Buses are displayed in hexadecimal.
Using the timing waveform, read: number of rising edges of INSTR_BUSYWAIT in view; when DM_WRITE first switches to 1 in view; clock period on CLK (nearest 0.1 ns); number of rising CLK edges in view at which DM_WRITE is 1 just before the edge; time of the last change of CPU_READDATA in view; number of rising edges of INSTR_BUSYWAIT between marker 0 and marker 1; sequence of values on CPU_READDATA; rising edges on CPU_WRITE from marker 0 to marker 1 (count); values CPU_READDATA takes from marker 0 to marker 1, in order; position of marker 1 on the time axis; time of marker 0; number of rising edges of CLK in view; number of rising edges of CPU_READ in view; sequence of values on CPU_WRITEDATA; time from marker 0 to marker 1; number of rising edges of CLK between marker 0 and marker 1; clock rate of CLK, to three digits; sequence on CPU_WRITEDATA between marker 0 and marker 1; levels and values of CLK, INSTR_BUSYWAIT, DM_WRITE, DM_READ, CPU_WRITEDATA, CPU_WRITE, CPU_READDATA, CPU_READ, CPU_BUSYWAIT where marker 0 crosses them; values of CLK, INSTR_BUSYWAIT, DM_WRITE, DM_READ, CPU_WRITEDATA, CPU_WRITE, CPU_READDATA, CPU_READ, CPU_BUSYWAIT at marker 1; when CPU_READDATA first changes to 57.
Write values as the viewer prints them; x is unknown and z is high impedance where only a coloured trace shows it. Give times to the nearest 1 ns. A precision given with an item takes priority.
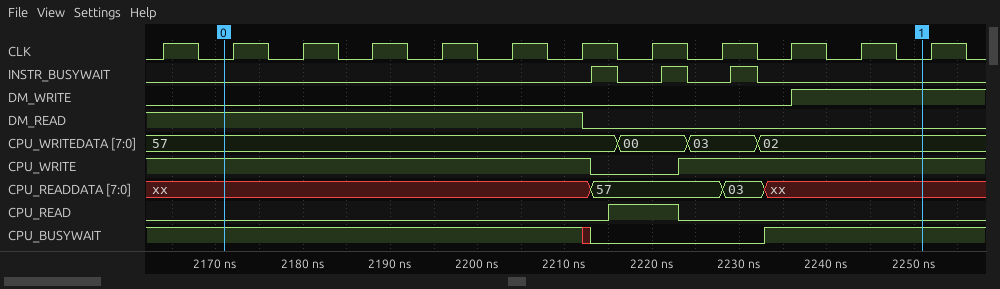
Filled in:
3
2236 ns
8 ns
2
2233 ns
3
xx, 57, 03, xx
1
xx, 57, 03, xx
2251 ns
2171 ns
12
1
57, 00, 03, 02
80 ns
10
125 MHz
57, 00, 03, 02
CLK=0, INSTR_BUSYWAIT=0, DM_WRITE=0, DM_READ=1, CPU_WRITEDATA=57, CPU_WRITE=1, CPU_READDATA=xx, CPU_READ=0, CPU_BUSYWAIT=1
CLK=0, INSTR_BUSYWAIT=0, DM_WRITE=1, DM_READ=0, CPU_WRITEDATA=02, CPU_WRITE=1, CPU_READDATA=xx, CPU_READ=0, CPU_BUSYWAIT=1
2213 ns
